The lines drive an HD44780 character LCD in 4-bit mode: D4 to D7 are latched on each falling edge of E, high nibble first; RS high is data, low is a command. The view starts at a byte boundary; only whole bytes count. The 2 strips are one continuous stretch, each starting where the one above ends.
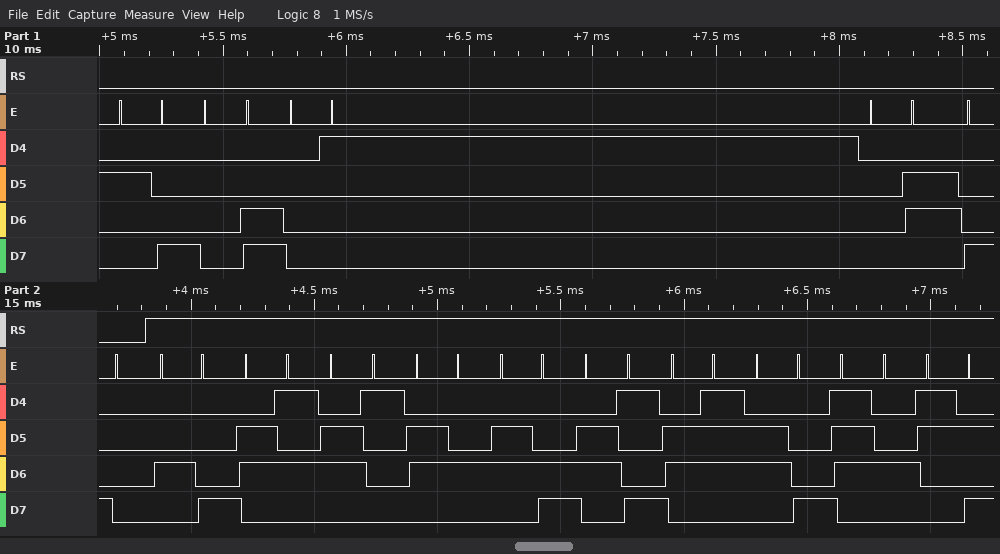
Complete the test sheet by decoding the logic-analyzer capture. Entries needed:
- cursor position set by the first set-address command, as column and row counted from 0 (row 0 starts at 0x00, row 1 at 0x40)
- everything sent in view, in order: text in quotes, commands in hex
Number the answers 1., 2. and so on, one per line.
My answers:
1. column 0, row 0
2. 0x28 0x0C 0x01 0x06 0x80 "Headlight:"
